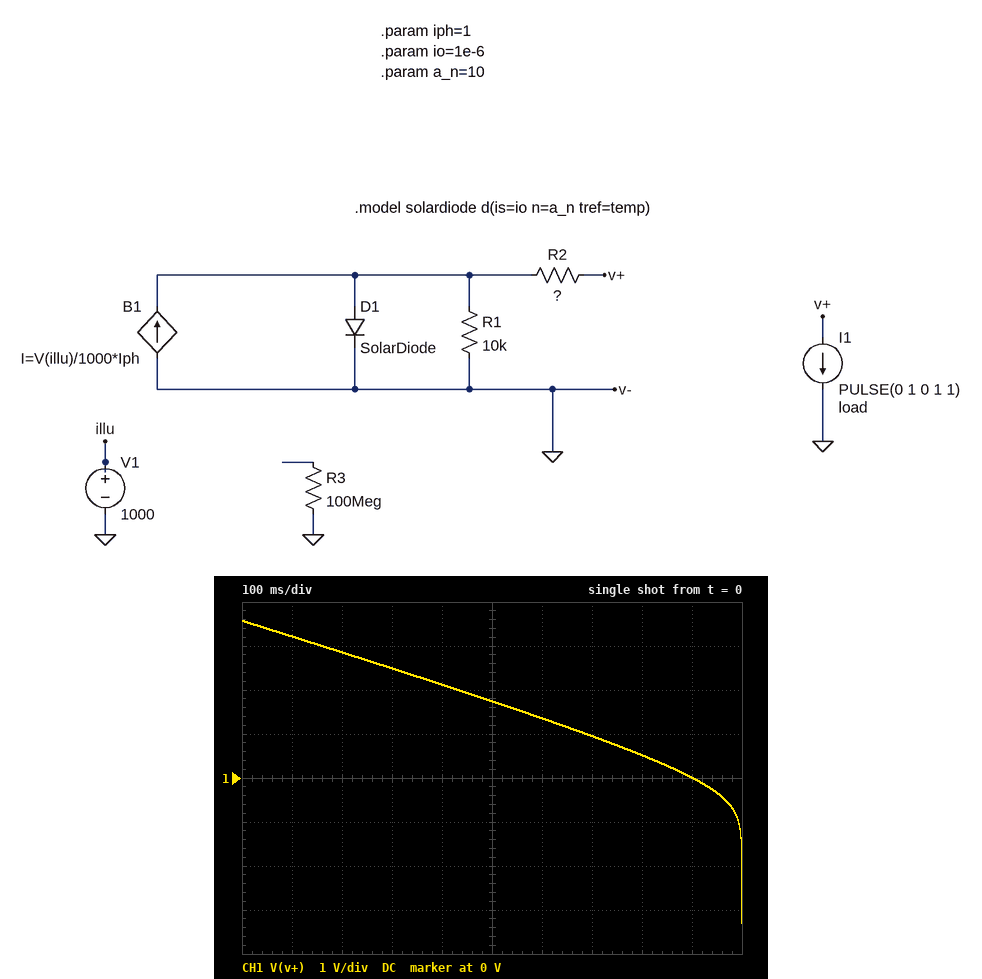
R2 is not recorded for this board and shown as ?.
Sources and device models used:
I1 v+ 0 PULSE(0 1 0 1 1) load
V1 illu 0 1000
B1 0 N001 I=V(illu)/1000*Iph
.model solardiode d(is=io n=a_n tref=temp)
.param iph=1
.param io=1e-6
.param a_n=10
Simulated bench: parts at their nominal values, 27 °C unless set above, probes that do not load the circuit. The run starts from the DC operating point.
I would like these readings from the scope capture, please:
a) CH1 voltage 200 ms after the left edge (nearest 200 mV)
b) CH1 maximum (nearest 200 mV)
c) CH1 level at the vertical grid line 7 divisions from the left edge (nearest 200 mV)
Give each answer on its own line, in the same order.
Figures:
2.8 V
3.6 V
1.0 V
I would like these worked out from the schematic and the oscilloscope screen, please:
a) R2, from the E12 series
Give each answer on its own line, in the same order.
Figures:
3.3 Ω
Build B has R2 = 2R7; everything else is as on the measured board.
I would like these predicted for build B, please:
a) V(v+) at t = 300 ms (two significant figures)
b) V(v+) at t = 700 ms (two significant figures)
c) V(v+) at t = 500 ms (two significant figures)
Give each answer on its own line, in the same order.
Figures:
2.7 V
1.4 V
2.0 V
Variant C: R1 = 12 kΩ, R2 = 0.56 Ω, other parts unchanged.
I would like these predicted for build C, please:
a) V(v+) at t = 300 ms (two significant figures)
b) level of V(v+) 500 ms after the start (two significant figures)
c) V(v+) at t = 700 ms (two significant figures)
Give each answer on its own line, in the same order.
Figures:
3.3 V
3.1 V
2.9 V
